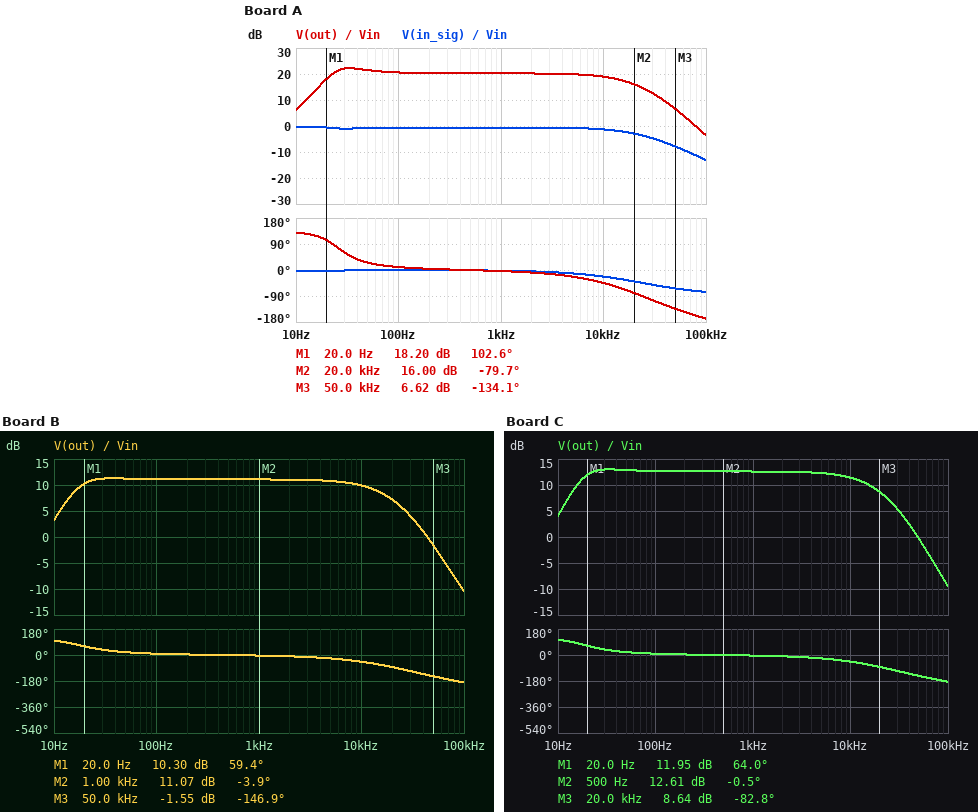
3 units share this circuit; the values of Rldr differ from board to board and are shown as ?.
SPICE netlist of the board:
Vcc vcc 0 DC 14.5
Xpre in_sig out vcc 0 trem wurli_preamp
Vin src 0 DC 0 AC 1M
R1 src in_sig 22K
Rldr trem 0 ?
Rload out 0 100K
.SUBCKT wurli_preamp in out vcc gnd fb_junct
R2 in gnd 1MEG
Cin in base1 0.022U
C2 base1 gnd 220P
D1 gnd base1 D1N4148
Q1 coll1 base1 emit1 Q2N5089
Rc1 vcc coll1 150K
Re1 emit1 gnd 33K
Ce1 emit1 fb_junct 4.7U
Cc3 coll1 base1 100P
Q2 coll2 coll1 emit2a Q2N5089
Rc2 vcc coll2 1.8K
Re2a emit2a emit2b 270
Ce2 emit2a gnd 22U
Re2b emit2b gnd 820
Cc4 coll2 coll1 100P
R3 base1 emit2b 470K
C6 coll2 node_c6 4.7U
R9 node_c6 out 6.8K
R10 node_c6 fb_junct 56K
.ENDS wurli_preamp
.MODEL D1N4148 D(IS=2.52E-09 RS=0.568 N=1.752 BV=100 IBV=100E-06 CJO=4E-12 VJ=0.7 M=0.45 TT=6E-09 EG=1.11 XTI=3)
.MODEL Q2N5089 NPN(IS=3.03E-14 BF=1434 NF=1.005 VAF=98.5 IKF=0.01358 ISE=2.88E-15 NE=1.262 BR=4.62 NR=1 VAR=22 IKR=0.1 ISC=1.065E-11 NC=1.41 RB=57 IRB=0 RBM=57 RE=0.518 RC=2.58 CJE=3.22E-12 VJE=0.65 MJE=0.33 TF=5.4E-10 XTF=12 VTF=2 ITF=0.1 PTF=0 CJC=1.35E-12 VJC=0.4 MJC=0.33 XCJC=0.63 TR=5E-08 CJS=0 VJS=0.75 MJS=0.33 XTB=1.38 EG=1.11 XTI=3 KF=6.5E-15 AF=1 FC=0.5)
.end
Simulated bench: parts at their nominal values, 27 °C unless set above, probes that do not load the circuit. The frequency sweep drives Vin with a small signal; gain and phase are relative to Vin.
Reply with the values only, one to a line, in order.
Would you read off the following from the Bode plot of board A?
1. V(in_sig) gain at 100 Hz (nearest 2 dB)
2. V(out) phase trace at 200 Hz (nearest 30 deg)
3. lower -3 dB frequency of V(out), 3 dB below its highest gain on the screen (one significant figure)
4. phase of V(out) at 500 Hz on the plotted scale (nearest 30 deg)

0 dB
0 deg
20 Hz
0 deg
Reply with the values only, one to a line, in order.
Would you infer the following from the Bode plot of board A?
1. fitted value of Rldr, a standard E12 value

5.6 kΩ
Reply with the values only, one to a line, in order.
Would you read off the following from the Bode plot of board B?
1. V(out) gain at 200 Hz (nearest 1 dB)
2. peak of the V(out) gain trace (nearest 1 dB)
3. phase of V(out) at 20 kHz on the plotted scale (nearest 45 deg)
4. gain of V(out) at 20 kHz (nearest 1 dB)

11 dB
11 dB
-90 deg
7 dB
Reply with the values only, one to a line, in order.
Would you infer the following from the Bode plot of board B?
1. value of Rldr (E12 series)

33 kΩ
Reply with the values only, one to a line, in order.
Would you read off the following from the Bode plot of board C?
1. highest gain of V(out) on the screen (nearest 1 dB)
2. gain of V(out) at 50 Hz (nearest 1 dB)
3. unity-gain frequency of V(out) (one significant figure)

13 dB
13 dB
50 kHz
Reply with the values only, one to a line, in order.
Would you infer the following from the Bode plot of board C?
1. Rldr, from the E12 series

22 kΩ
